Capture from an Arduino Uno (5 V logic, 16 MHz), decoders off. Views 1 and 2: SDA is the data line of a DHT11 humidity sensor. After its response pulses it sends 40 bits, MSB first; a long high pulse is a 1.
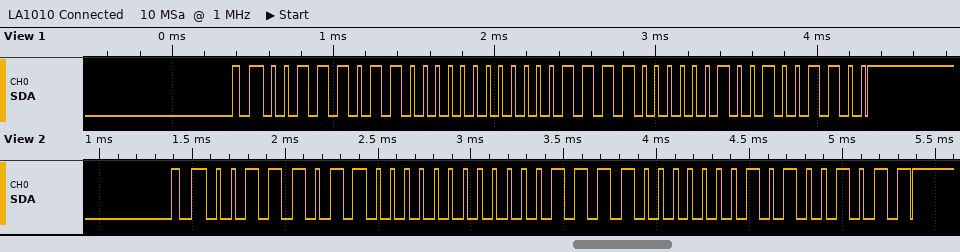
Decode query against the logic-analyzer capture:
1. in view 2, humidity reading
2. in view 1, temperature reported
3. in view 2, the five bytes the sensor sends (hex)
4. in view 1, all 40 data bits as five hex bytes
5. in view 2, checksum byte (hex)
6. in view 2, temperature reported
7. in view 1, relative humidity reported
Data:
59 %
15.2 °C
3B 00 0F 01 4B
3B 00 0F 02 4C
0x4B
15.1 °C
59 %
